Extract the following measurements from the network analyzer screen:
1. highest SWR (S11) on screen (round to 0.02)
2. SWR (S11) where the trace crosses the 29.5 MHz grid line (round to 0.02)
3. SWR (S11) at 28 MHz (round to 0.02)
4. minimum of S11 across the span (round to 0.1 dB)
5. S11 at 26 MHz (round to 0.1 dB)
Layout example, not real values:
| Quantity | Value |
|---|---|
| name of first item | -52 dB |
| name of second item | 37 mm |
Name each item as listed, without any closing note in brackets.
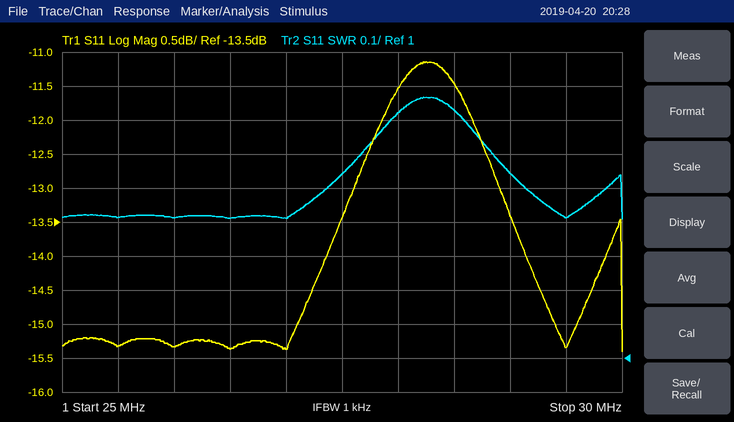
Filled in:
| Quantity | Value |
|---|---|
| highest SWR (S11) on screen | 1.76 |
| SWR (S11) where the trace crosses the 29.5 MHz grid line | 1.42 |
| SWR (S11) at 28 MHz | 1.72 |
| minimum of S11 across the span | -15.4 dB |
| S11 at 26 MHz | -15.3 dB |
